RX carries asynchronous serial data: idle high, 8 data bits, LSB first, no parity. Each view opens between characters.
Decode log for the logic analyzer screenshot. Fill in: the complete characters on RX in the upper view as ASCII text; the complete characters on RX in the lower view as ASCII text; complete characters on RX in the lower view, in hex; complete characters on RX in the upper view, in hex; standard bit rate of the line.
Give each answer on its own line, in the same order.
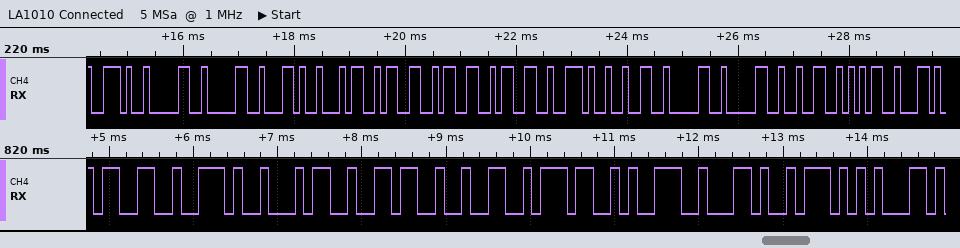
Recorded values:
".00,4333.20025"
"3.46279,W"
33, 2E, 34, 36, 32, 37, 39, 2C, 57
2E, 30, 30, 2C, 34, 33, 33, 33, 2E, 32, 30, 30, 32, 35
9600 baud
